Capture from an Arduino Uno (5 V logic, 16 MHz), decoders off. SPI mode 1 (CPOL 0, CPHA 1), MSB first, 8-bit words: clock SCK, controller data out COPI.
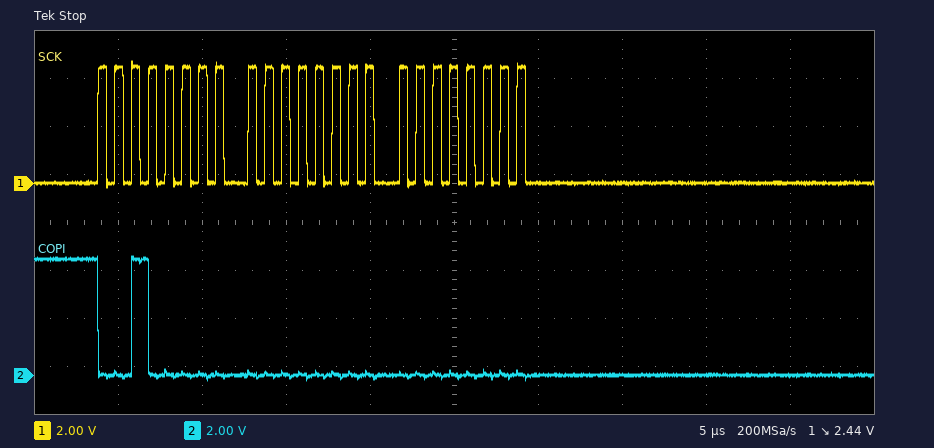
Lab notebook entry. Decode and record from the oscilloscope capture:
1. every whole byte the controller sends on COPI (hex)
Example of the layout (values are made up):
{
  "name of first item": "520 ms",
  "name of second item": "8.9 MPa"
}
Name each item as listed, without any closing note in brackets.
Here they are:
{
  "every whole byte the controller sends on COPI": "20 00 00"
}
